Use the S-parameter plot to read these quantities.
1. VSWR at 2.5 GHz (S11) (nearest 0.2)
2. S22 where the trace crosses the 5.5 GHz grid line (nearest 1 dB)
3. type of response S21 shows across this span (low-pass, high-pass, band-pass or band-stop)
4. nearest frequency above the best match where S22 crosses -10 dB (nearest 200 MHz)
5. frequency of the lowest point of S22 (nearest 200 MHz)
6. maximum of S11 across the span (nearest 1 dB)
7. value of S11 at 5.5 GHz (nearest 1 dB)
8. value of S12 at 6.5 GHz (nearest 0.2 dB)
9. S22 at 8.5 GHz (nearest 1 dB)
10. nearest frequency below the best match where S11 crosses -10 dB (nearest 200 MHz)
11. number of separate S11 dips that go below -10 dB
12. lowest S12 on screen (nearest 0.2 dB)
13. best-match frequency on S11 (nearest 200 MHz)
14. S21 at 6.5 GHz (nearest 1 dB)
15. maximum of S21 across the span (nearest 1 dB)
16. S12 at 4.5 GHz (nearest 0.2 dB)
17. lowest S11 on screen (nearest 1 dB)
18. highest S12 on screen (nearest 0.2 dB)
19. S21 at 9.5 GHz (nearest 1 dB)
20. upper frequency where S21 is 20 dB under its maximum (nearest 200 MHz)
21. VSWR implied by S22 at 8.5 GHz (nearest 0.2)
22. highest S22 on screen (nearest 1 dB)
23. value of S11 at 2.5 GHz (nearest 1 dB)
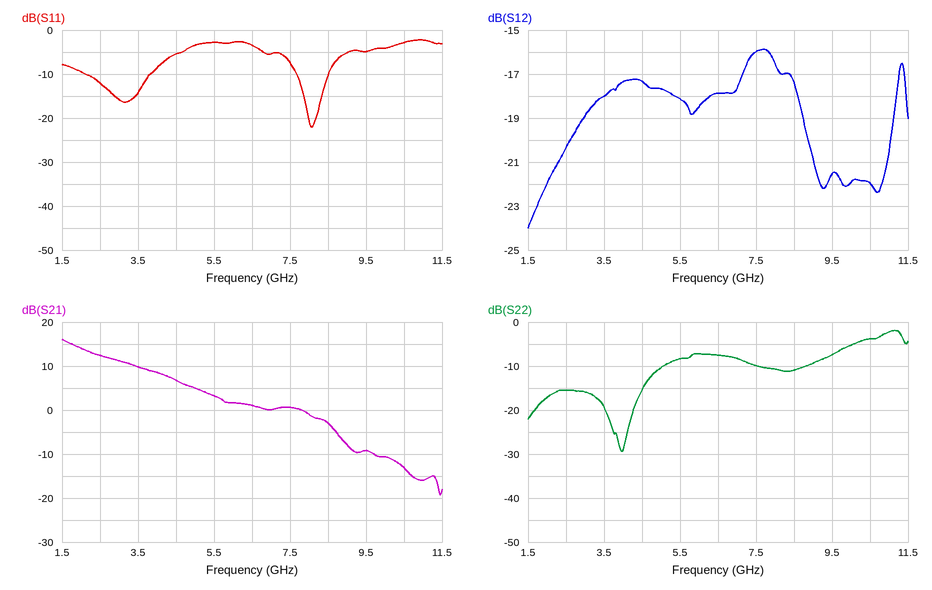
1.6
-8 dB
low-pass
5.0 GHz
4.0 GHz
-2 dB
-3 dB
-17.8 dB
-11 dB
7.6 GHz
2
-24.0 dB
8.0 GHz
1 dB
16 dB
-17.4 dB
-22 dB
-15.8 dB
-9 dB
8.6 GHz
1.8
-2 dB
-12 dB
